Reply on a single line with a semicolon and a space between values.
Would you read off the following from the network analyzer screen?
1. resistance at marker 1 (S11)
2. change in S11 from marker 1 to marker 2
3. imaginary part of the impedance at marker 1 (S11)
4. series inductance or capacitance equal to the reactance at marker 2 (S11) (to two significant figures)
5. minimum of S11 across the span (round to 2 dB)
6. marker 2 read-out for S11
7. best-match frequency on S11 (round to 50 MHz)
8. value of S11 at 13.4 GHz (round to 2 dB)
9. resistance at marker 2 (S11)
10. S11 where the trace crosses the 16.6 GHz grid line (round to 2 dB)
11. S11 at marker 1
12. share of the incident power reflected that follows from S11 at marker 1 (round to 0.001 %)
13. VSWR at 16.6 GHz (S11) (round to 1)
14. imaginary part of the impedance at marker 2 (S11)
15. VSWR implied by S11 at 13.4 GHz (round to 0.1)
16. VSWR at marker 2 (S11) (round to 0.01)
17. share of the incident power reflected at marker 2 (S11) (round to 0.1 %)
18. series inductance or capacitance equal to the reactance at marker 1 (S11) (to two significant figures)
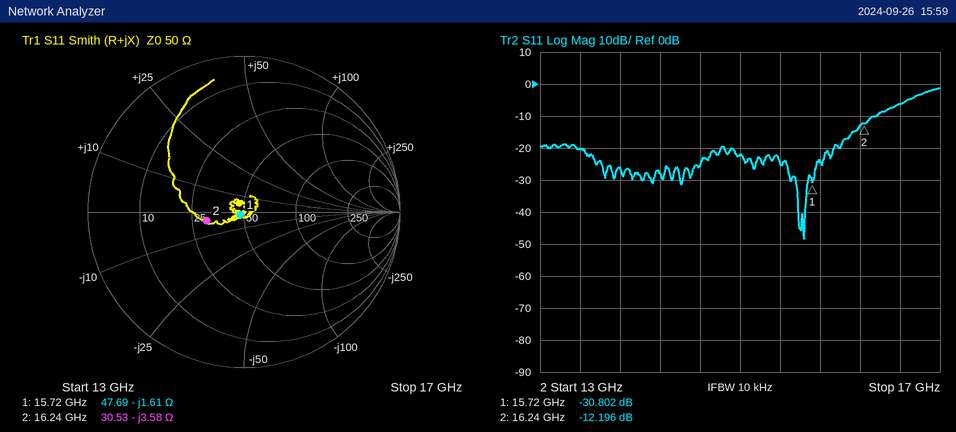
47.69 Ω; 18.606 dB; -1.61 Ω; 2.7 pF; -48 dB; -12.196 dB; 15.65 GHz; -20 dB; 30.53 Ω; -6 dB; -30.802 dB; 0.083 %; 3; -3.58 Ω; 1.2; 1.65; 6.0 %; 6.3 pF
